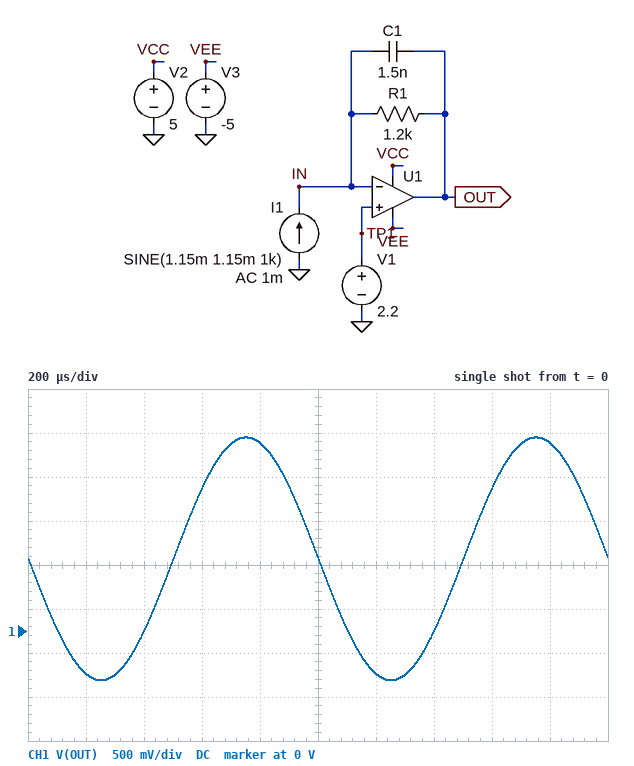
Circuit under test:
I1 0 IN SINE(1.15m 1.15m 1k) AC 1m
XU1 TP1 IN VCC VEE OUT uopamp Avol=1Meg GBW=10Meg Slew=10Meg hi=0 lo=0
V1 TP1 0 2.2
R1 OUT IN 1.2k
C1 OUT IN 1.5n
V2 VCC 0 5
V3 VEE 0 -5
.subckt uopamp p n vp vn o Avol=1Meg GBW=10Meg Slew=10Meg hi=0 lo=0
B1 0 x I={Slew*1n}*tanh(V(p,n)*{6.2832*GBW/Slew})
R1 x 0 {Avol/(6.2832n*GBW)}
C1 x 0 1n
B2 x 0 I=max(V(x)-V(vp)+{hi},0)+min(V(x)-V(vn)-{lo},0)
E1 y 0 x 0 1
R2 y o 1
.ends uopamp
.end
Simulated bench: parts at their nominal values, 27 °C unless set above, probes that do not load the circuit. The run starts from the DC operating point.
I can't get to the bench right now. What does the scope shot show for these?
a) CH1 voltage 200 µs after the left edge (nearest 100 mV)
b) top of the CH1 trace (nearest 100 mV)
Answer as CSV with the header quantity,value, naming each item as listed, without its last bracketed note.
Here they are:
quantity,value
CH1 voltage 200 µs after the left edge,-500 mV
top of the CH1 trace,2.2 V
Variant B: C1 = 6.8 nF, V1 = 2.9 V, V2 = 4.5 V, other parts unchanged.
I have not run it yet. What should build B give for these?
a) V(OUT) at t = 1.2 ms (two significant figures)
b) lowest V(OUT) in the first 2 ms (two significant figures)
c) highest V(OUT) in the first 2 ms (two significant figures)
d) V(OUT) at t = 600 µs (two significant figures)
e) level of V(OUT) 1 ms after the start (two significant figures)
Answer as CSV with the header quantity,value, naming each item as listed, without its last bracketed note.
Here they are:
quantity,value
V(OUT) at t = 1.2 ms,230 mV
lowest V(OUT) in the first 2 ms,140 mV
highest V(OUT) in the first 2 ms,2.9 V
V(OUT) at t = 600 µs,2.3 V
level of V(OUT) 1 ms after the start,1.6 V
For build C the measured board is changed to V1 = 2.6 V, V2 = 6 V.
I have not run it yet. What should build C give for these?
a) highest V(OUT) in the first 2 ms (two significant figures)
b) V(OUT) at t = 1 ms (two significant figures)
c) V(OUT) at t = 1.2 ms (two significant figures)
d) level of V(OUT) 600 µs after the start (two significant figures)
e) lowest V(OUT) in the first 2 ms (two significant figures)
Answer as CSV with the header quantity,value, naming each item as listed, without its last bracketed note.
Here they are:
quantity,value
highest V(OUT) in the first 2 ms,2.6 V
V(OUT) at t = 1 ms,1.2 V
V(OUT) at t = 1.2 ms,-87 mV
level of V(OUT) 600 µs after the start,2.0 V
lowest V(OUT) in the first 2 ms,-160 mV
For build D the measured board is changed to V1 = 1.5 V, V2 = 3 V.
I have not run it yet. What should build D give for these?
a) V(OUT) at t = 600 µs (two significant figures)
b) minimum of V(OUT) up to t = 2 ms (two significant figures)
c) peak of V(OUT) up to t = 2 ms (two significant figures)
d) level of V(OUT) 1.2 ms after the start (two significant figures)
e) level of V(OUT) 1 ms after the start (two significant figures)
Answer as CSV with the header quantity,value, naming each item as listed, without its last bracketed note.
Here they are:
quantity,value
V(OUT) at t = 600 µs,920 mV
minimum of V(OUT) up to t = 2 ms,-1.3 V
peak of V(OUT) up to t = 2 ms,1.5 V
level of V(OUT) 1.2 ms after the start,-1.2 V
level of V(OUT) 1 ms after the start,140 mV
